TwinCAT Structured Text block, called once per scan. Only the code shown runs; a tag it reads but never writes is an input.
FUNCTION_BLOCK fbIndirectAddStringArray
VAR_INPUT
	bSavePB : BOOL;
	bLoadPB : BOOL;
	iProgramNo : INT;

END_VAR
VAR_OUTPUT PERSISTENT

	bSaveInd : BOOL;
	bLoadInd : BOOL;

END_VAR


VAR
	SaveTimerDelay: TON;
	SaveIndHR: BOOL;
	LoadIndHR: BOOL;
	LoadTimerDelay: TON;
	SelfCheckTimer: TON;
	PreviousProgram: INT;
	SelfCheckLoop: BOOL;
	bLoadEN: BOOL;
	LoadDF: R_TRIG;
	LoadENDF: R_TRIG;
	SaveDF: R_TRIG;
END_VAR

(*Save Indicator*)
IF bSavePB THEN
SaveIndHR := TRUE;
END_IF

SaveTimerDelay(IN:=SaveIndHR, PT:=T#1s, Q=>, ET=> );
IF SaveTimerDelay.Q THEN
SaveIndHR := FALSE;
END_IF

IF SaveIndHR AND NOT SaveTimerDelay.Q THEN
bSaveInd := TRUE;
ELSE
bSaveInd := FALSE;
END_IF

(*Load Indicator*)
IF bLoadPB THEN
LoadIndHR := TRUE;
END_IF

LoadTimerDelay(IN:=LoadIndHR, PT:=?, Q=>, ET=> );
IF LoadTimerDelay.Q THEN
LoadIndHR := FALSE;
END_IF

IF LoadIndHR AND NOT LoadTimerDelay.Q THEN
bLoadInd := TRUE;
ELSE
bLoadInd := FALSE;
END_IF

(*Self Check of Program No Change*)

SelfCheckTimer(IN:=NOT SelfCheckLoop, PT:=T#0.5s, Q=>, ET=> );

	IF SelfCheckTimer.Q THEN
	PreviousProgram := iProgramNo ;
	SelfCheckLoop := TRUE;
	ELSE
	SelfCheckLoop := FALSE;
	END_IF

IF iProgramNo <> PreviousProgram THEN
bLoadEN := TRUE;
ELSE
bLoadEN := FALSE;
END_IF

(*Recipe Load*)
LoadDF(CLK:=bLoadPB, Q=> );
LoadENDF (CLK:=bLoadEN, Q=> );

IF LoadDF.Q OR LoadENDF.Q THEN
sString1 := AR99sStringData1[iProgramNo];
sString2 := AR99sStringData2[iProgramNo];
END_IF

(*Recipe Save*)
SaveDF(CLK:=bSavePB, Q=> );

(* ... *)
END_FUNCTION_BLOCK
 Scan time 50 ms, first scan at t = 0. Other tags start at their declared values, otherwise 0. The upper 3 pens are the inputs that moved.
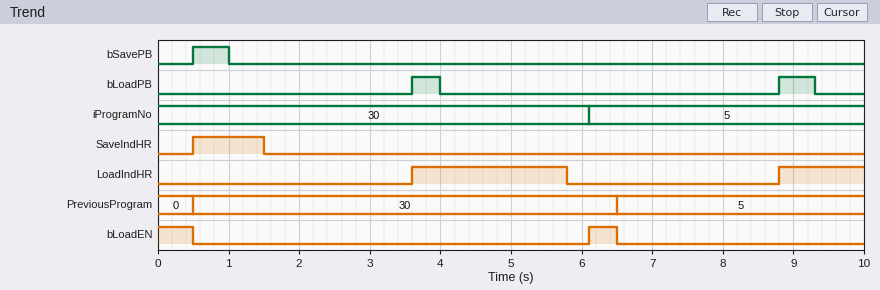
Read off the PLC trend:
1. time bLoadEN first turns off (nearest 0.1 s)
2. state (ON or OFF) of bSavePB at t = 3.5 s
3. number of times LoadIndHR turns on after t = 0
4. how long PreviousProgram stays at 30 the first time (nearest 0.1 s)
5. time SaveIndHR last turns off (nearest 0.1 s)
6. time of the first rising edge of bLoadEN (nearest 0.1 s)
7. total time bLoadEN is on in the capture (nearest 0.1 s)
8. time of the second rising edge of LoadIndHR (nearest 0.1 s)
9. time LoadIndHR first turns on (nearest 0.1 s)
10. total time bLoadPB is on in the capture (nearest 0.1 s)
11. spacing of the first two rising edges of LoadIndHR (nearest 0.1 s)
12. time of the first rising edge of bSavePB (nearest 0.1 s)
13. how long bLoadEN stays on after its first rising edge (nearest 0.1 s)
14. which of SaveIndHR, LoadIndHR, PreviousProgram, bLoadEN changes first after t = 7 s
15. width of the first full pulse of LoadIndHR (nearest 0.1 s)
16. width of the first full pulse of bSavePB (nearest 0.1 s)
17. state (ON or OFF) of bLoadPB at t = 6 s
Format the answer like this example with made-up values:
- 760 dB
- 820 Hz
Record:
- 0.5 s
- OFF
- 2
- 6.0 s
- 1.5 s
- 6.1 s
- 0.9 s
- 8.8 s
- 3.6 s
- 0.9 s
- 5.2 s
- 0.5 s
- 0.4 s
- LoadIndHR
- 2.2 s
- 0.5 s
- OFF
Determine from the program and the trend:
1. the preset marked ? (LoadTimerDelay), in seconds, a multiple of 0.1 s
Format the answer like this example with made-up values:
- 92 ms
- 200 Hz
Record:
- 2.2 s
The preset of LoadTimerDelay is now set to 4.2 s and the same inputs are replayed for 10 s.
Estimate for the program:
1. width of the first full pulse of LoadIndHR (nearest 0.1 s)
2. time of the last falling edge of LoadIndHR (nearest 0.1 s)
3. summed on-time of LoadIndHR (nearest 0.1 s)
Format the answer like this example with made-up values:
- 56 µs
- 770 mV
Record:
- 4.2 s
- 7.8 s
- 5.4 s
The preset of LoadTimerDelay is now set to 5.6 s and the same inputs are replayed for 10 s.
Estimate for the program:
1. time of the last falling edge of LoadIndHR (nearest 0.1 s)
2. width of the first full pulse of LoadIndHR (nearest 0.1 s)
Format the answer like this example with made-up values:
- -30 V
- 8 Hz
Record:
- 9.2 s
- 5.6 s
